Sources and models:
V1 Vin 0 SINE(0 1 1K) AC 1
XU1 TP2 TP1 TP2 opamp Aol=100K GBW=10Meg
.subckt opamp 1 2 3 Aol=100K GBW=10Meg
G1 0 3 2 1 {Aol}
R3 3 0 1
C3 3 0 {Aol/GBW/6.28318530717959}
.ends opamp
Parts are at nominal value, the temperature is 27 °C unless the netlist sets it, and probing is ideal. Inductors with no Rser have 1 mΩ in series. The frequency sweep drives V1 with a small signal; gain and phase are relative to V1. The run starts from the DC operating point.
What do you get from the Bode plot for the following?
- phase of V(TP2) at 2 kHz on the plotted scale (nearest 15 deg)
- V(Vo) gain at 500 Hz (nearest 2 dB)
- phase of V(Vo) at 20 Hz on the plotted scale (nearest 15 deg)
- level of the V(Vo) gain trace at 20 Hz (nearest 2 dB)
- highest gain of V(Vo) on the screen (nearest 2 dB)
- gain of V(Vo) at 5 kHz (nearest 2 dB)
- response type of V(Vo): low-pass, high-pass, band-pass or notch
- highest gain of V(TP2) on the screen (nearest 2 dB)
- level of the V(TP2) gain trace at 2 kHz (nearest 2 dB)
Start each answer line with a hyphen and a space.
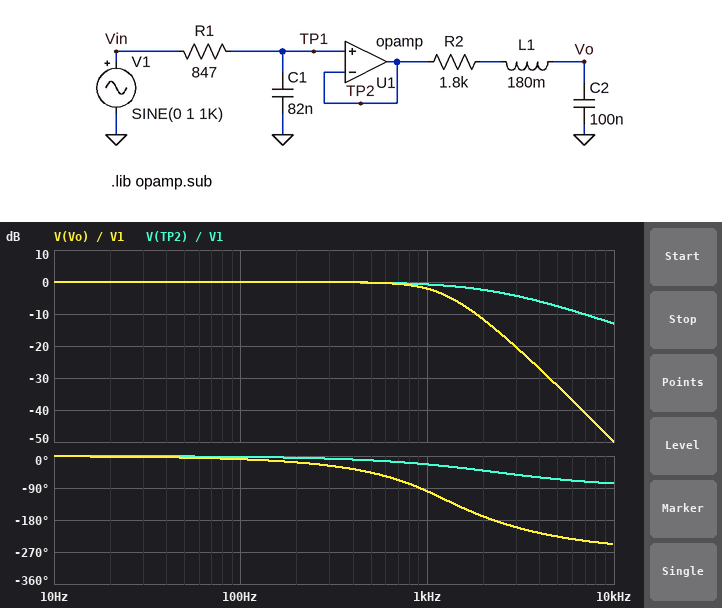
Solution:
- -45 deg
- 0 dB
- 0 deg
- 0 dB
- 0 dB
- -32 dB
- low-pass
- 0 dB
- -2 dB
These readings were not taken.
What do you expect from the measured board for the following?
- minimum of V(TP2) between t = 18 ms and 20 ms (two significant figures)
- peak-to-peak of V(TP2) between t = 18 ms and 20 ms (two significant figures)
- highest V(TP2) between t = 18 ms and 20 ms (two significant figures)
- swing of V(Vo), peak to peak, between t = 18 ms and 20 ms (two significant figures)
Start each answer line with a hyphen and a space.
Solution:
- -920 mV
- 1.8 V
- 920 mV
- 1.6 V
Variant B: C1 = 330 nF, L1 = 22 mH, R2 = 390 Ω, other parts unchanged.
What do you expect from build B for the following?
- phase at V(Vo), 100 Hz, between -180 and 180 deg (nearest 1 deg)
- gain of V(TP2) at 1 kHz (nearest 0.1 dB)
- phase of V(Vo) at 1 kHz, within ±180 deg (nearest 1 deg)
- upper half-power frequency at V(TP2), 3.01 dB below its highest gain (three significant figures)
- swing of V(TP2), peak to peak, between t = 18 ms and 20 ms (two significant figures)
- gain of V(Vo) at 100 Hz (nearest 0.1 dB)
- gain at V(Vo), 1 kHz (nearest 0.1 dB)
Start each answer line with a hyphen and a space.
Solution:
- -11 deg
- -6.1 dB
- -75 deg
- 569 Hz
- 990 mV
- -0.1 dB
- -5.6 dB
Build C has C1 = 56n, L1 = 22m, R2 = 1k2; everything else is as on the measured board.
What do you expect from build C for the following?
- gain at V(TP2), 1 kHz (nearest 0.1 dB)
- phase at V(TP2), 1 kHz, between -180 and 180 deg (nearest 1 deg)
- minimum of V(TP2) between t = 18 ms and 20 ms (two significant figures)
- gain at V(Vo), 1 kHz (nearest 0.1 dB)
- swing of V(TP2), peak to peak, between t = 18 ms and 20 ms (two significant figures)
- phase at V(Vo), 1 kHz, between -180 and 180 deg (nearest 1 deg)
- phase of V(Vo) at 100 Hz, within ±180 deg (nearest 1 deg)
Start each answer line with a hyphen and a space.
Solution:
- -0.4 dB
- -17 deg
- -960 mV
- -1.8 dB
- 1.9 V
- -56 deg
- -6 deg
